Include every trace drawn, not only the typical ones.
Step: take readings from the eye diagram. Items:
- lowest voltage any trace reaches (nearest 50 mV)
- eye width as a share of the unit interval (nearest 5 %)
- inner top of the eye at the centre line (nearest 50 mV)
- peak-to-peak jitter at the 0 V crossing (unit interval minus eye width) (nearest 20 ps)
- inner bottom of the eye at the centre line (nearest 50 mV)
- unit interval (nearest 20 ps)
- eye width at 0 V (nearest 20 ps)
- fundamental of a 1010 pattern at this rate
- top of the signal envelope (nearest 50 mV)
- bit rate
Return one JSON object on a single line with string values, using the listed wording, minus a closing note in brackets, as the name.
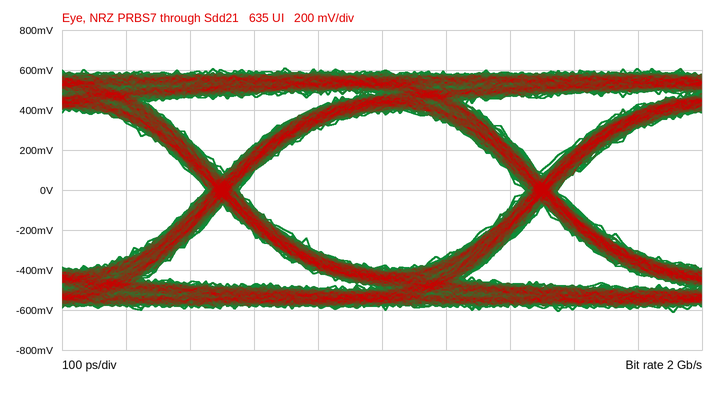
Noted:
{"lowest voltage any trace reaches": "-600 mV", "eye width as a share of the unit interval": "90 %", "inner top of the eye at the centre line": "400 mV", "peak-to-peak jitter at the 0 V crossing (unit interval minus eye width)": "60 ps", "inner bottom of the eye at the centre line": "-400 mV", "unit interval": "500 ps", "eye width at 0 V": "440 ps", "fundamental of a 1010 pattern at this rate": "1 GHz", "top of the signal envelope": "600 mV", "bit rate": "2 Gb/s"}
